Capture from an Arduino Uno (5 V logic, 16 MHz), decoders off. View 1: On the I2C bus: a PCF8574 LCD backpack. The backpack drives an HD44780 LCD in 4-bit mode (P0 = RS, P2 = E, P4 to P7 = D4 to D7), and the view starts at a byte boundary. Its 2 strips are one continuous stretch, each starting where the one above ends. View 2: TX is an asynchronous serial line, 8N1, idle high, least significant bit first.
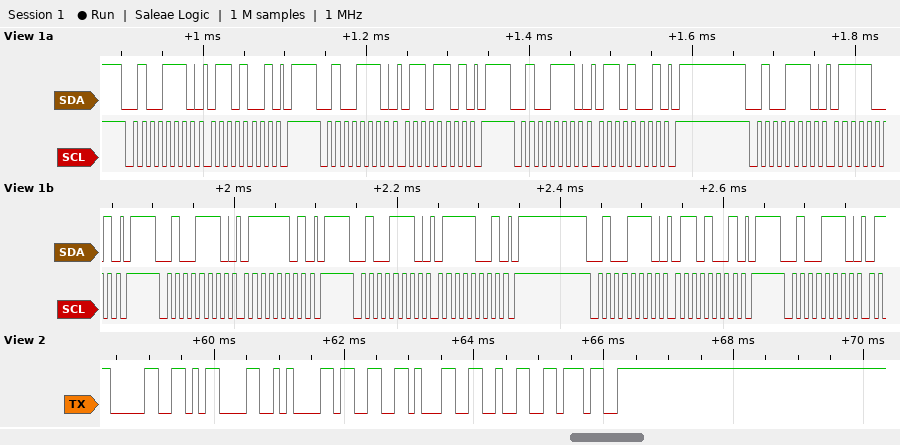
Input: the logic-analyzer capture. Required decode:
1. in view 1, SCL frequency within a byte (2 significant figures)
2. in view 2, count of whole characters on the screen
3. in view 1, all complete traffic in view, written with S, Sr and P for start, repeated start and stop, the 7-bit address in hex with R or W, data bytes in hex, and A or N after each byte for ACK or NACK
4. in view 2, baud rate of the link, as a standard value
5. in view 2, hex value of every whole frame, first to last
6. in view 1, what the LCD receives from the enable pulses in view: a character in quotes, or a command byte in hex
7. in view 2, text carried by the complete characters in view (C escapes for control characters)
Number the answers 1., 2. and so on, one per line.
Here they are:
1. 100 kHz
2. 7
3. S 27W A 69 A P S 27W A 6D A P S 27W A 69 A P S 27W A 79 A P S 27W A 7D A P S 27W A 79 A P S 27W A 69 A P S 27W A
4. 9600 baud
5. 30 0D 0A 33 31 32 37
6. 'g'
7. "0\r\n3127"
